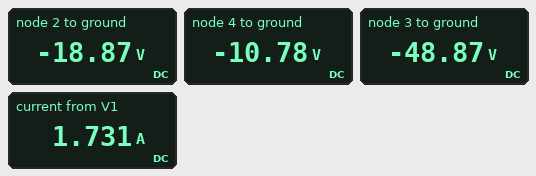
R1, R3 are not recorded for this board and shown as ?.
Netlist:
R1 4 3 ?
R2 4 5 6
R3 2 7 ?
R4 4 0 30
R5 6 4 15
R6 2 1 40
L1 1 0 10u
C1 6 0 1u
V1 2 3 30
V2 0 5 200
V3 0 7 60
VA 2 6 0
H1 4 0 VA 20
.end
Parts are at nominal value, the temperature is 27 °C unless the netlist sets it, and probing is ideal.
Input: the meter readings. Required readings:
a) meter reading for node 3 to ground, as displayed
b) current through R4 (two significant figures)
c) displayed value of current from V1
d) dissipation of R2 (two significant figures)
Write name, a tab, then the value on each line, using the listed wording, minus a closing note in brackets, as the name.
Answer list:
meter reading for node 3 to ground, as displayed	-48.87 V
current through R4	360 mA
displayed value of current from V1	1.731 A
dissipation of R2	6.0 kW
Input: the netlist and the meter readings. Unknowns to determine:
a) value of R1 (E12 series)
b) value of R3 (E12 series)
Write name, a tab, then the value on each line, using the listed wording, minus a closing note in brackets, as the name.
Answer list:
value of R1	22 Ω
value of R3	15 Ω
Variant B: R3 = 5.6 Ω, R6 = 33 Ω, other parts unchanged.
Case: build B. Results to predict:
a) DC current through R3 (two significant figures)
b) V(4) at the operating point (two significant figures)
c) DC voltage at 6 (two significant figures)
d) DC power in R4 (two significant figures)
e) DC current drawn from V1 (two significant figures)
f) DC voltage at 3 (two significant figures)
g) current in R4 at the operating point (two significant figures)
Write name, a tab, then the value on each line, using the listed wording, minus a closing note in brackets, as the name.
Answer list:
DC current through R3	4.2 A
V(4) at the operating point	-21 V
DC voltage at 6	-36 V
DC power in R4	14 W
DC current drawn from V1	2.1 A
DC voltage at 3	-66 V
current in R4 at the operating point	690 mA
